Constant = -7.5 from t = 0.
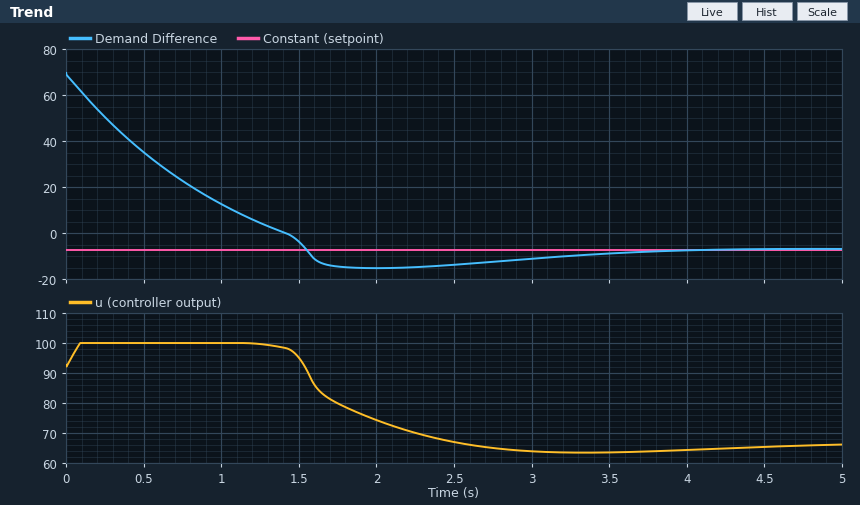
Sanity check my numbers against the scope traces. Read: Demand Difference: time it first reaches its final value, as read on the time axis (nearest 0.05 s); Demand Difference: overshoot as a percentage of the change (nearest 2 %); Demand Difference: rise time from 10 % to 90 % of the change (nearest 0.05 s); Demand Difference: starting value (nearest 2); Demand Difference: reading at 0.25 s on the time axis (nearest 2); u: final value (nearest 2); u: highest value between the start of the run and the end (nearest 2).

1.55 s
10 %
1.30 s
70
50
66
100
